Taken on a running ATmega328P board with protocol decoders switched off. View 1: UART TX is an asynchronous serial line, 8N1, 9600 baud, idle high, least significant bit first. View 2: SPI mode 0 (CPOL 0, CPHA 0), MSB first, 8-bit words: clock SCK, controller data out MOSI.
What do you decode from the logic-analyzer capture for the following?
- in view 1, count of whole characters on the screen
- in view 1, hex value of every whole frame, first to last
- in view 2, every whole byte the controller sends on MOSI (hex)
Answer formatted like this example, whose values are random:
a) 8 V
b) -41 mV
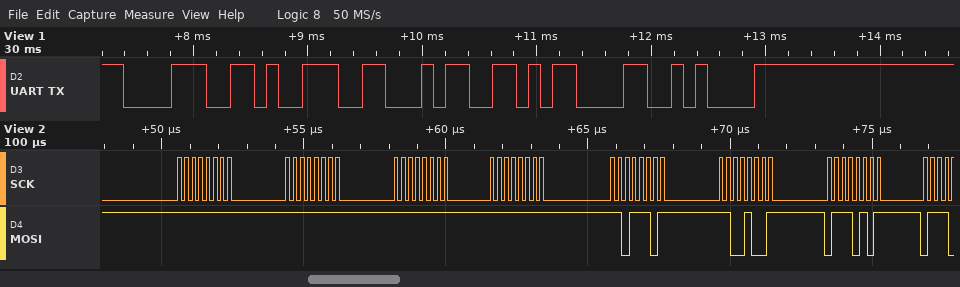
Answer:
a) 5
b) 38 39 34 0D 0A
c) FF FF FF FF DD C9 75
